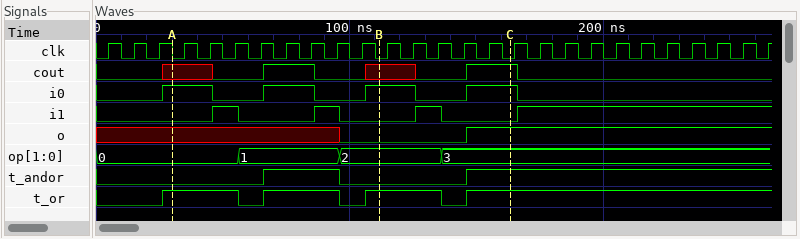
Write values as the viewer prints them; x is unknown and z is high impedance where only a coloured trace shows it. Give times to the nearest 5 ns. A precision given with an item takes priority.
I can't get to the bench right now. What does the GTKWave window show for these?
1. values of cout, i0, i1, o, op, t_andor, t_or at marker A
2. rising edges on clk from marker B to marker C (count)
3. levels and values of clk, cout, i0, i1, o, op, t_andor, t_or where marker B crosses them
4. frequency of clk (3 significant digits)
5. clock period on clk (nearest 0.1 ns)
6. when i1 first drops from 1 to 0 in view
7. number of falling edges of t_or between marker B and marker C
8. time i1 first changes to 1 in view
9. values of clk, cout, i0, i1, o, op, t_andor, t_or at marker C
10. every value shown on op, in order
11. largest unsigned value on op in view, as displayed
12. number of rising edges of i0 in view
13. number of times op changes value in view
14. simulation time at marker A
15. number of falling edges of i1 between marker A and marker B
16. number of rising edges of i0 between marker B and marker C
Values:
cout=x, i0=1, i1=0, o=x, op=0, t_andor=0, t_or=1
5
clk=0, cout=x, i0=1, i1=0, o=0, op=2, t_andor=0, t_or=1
100 MHz
10 ns
55 ns
1
45 ns
clk=0, cout=1, i0=1, i1=0, o=1, op=3, t_andor=1, t_or=1
0, 1, 2, 3
3
4
3
30 ns
2
1
